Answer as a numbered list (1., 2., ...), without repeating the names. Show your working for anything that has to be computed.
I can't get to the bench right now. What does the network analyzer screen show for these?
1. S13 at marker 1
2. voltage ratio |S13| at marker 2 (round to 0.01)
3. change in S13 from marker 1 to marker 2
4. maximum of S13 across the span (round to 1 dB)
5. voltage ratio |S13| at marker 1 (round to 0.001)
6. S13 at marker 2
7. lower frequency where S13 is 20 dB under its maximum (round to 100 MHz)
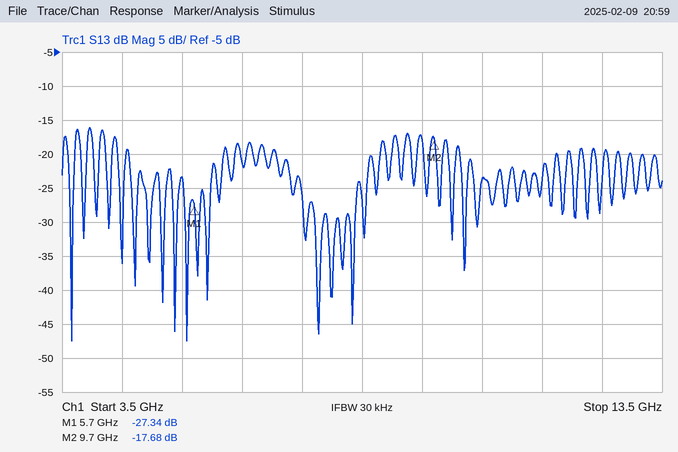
1. -27.34 dB
2. 10^(-17.68/20) ≈ 0.13
3. -17.68 − (-27.34) = 9.66 dB
4. -16 dB
5. 10^(-27.34/20) ≈ 0.043
6. -17.68 dB
7. 3.7 GHz
